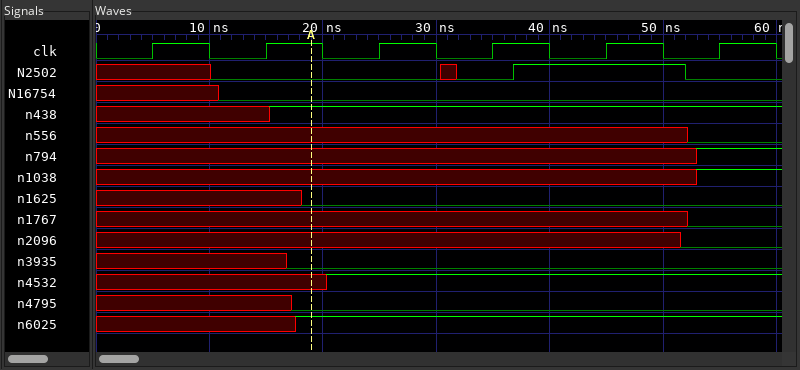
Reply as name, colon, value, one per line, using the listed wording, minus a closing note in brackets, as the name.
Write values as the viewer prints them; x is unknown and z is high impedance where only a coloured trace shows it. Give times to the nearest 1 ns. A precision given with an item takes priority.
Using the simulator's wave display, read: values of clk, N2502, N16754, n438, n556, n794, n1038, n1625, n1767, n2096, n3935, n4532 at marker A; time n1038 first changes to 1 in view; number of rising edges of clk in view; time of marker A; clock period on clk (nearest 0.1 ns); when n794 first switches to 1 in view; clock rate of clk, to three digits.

values of clk, N2502, N16754, n438, n556, n794, n1038, n1625, n1767, n2096, n3935, n4532 at marker A: clk=1, N2502=0, N16754=0, n438=1, n556=x, n794=x, n1038=x, n1625=0, n1767=x, n2096=x, n3935=0, n4532=x
time n1038 first changes to 1 in view: 53 ns
number of rising edges of clk in view: 6
time of marker A: 19 ns
clock period on clk: 10 ns
when n794 first switches to 1 in view: 53 ns
clock rate of clk, to three digits: 100 MHz
